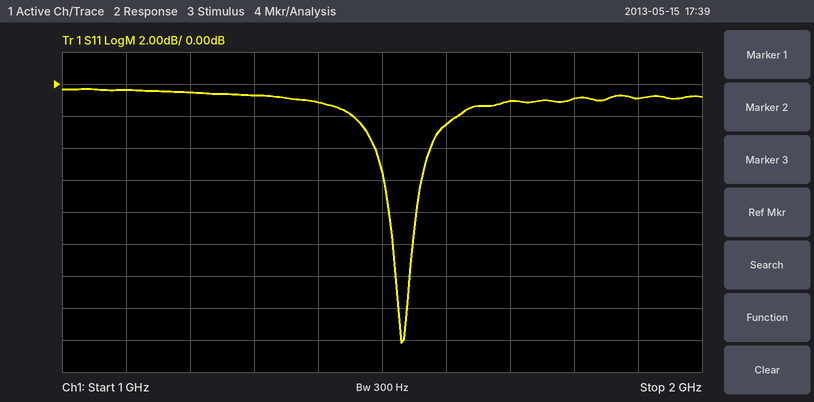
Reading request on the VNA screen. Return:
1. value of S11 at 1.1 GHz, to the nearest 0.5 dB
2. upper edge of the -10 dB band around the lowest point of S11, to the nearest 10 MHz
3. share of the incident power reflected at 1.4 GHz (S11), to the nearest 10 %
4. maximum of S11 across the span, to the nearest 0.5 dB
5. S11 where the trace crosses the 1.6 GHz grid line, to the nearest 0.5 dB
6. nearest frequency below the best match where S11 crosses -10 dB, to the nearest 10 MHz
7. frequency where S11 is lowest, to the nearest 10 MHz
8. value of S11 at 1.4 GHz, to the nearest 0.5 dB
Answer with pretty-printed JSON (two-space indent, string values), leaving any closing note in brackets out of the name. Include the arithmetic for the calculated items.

{
  "value of S11 at 1.1 GHz, to the nearest 0.5 dB": "-0.5 dB",
  "upper edge of the -10 dB band around the lowest point of S11, to the nearest 10 MHz": "1.55 GHz",
  "share of the incident power reflected at 1.4 GHz (S11), to the nearest 10 %": "10^(-1/10) ≈ 79.4 %, so 80 % to the nearest 10 %",
  "maximum of S11 across the span, to the nearest 0.5 dB": "-0.5 dB",
  "S11 where the trace crosses the 1.6 GHz grid line, to the nearest 0.5 dB": "-2.5 dB",
  "nearest frequency below the best match where S11 crosses -10 dB, to the nearest 10 MHz": "1.52 GHz",
  "frequency where S11 is lowest, to the nearest 10 MHz": "1.53 GHz",
  "value of S11 at 1.4 GHz, to the nearest 0.5 dB": "-1.0 dB"
}
